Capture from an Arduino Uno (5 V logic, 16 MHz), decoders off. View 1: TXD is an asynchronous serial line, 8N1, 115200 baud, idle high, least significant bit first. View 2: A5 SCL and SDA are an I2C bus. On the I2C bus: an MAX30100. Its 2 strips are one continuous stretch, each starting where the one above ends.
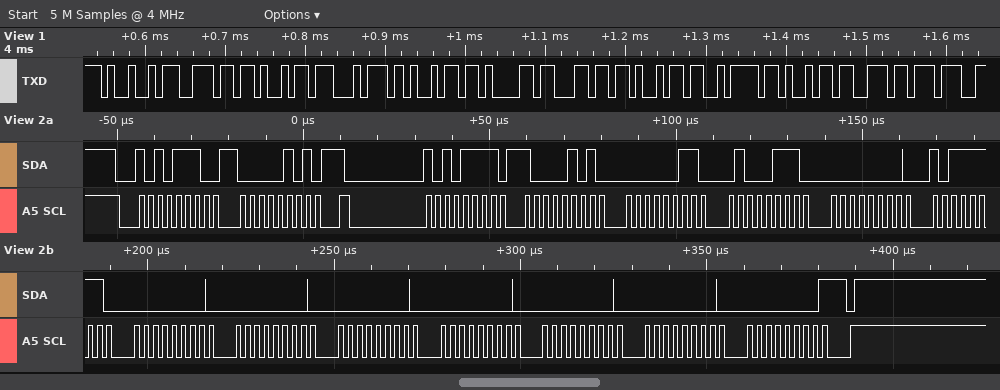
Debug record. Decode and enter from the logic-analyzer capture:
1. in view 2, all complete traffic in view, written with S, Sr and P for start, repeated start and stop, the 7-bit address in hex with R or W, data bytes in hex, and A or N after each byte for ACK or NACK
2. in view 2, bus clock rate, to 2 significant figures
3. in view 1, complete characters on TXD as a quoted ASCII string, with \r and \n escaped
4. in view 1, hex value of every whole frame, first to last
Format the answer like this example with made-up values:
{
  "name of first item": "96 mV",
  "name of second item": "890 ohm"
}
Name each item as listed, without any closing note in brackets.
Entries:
{
  "in view 2, all complete traffic in view, written with S, Sr and P for start, repeated start and stop, the 7-bit address in hex with R or W, data bytes in hex, and A or N after each byte for ACK or NACK": "S 57W A 05 A Sr 57R A 85 A 03 A 47 A 00 A BF A 00 A 00 A 00 A 00 A 00 A 00 A 00 N P",
  "in view 2, bus clock rate, to 2 significant figures": "400 kHz",
  "in view 1, complete characters on TXD as a quoted ASCII string, with \\r and \\n escaped": "\"Initializin\"",
  "in view 1, hex value of every whole frame, first to last": "49 6E 69 74 69 61 6C 69 7A 69 6E"
}
